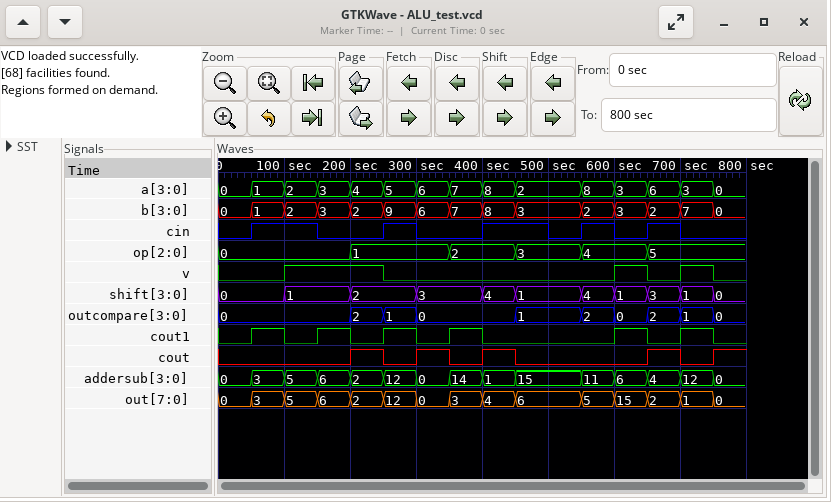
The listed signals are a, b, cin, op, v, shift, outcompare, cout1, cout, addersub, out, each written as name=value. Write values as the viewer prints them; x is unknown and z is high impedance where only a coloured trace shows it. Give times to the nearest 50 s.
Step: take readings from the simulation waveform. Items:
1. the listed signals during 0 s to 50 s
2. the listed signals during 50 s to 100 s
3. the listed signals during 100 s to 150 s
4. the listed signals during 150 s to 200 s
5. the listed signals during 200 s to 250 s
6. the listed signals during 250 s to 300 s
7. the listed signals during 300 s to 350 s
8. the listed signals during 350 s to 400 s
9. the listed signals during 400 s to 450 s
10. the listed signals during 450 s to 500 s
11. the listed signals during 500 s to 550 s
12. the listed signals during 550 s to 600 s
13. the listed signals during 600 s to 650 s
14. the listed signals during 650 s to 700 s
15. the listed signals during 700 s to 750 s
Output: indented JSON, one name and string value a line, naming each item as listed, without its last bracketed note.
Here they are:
{
  "the listed signals during 0 s to 50 s": "a=0, b=0, cin=0, op=0, v=0, shift=0, outcompare=0, cout1=0, cout=0, addersub=0, out=0",
  "the listed signals during 50 s to 100 s": "a=1, b=1, cin=1, op=0, v=0, shift=0, outcompare=0, cout1=1, cout=0, addersub=3, out=3",
  "the listed signals during 100 s to 150 s": "a=2, b=2, cin=1, op=0, v=1, shift=1, outcompare=0, cout1=0, cout=0, addersub=5, out=5",
  "the listed signals during 150 s to 200 s": "a=3, b=3, cin=0, op=0, v=1, shift=1, outcompare=0, cout1=1, cout=0, addersub=6, out=6",
  "the listed signals during 200 s to 250 s": "a=4, b=2, cin=0, op=1, v=1, shift=2, outcompare=2, cout1=0, cout=1, addersub=2, out=2",
  "the listed signals during 250 s to 300 s": "a=5, b=9, cin=1, op=1, v=0, shift=2, outcompare=1, cout1=1, cout=0, addersub=12, out=12",
  "the listed signals during 300 s to 350 s": "a=6, b=6, cin=0, op=1, v=0, shift=3, outcompare=0, cout1=0, cout=1, addersub=0, out=0",
  "the listed signals during 350 s to 400 s": "a=7, b=7, cin=0, op=2, v=0, shift=3, outcompare=0, cout1=1, cout=0, addersub=14, out=3",
  "the listed signals during 400 s to 450 s": "a=8, b=8, cin=1, op=2, v=0, shift=4, outcompare=0, cout1=0, cout=1, addersub=1, out=4",
  "the listed signals during 450 s to 500 s": "a=2, b=3, cin=1, op=3, v=0, shift=1, outcompare=1, cout1=0, cout=0, addersub=15, out=6",
  "the listed signals during 500 s to 550 s": "a=2, b=3, cin=0, op=3, v=0, shift=1, outcompare=1, cout1=0, cout=0, addersub=15, out=6",
  "the listed signals during 550 s to 600 s": "a=8, b=2, cin=1, op=4, v=0, shift=4, outcompare=2, cout1=0, cout=0, addersub=11, out=5",
  "the listed signals during 600 s to 650 s": "a=3, b=3, cin=0, op=4, v=1, shift=1, outcompare=0, cout1=1, cout=0, addersub=6, out=15",
  "the listed signals during 650 s to 700 s": "a=6, b=2, cin=1, op=5, v=0, shift=3, outcompare=2, cout1=0, cout=1, addersub=4, out=2",
  "the listed signals during 700 s to 750 s": "a=3, b=7, cin=0, op=5, v=1, shift=1, outcompare=1, cout1=1, cout=0, addersub=12, out=1"
}
